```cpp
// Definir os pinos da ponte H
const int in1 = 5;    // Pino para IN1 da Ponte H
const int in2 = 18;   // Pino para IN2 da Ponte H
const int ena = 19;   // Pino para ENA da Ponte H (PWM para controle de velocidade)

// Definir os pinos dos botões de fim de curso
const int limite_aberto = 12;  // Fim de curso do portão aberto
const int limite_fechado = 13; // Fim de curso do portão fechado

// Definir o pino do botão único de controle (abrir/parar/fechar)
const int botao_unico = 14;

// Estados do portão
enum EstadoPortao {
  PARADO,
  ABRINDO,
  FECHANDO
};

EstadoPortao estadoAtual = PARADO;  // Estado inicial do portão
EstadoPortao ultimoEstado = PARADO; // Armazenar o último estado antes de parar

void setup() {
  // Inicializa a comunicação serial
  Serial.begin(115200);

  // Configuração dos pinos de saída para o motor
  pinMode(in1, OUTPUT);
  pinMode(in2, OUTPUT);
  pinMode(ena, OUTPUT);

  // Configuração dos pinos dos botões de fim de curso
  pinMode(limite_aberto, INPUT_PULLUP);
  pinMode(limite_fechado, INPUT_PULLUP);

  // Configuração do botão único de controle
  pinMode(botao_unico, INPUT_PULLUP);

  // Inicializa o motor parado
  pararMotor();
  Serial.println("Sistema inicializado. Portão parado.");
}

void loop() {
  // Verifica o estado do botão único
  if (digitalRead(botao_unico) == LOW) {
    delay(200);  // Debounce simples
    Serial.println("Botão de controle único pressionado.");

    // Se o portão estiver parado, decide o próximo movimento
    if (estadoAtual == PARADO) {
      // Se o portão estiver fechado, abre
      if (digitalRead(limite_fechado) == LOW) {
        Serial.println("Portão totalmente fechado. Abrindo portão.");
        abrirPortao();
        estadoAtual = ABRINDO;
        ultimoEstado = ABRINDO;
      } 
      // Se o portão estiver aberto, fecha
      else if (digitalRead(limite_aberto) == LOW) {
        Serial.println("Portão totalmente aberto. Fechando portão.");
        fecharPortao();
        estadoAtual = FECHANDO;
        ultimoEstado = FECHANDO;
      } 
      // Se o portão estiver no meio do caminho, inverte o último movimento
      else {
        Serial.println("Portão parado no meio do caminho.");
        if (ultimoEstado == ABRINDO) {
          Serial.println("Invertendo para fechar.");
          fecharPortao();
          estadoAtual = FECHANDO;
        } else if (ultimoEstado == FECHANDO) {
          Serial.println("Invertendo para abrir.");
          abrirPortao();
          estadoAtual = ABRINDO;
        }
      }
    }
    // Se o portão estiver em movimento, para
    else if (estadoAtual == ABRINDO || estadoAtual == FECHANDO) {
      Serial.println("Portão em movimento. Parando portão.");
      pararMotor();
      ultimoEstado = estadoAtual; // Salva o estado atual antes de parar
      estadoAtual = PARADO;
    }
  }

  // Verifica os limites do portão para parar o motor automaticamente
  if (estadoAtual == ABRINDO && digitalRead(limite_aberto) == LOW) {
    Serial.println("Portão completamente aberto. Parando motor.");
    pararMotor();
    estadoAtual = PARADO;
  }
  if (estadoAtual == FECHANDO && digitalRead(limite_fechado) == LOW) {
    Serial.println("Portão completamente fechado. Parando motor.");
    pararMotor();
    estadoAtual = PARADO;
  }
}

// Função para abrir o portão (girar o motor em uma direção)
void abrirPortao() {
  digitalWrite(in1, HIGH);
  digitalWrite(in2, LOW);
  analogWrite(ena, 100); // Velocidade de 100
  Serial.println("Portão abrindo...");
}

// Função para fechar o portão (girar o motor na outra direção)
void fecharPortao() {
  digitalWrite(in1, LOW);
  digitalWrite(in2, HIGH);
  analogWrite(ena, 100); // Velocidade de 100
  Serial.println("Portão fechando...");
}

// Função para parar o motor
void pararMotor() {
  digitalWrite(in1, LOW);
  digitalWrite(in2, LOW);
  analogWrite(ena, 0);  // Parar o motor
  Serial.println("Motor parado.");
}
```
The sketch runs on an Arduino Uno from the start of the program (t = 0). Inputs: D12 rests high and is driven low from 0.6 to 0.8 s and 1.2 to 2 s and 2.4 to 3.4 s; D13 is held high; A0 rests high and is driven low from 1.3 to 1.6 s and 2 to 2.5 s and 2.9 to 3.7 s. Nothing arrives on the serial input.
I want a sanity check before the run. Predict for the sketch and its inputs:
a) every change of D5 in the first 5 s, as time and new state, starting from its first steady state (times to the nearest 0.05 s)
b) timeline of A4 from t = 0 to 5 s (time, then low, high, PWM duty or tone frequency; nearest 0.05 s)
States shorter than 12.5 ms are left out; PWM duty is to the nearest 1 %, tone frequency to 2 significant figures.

0 s low; 2.2 s high; 2.4 s low; 3.7 s high
0 s low; 1.5 s high; 1.7 s low; 2.6 s high; 3.1 s low; 3.3 s high; 3.5 s low
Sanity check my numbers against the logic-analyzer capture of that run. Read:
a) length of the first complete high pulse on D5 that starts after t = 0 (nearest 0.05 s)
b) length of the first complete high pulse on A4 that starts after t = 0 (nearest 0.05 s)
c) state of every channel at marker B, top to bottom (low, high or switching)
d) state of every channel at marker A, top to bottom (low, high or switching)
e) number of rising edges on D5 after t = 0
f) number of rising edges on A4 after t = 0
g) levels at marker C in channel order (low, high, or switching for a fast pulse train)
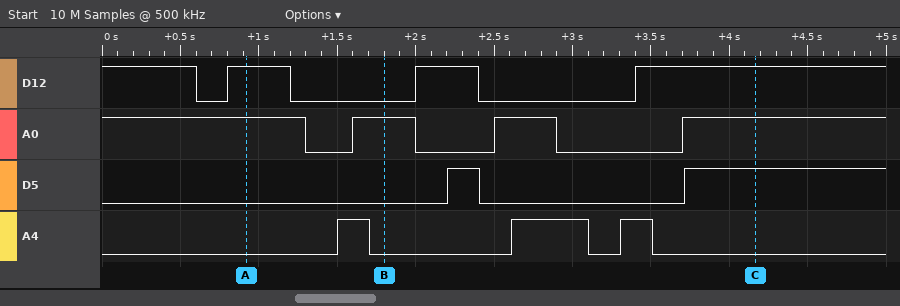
0.20 s
0.20 s
D12 low, A0 high, D5 low, A4 low
D12 high, A0 high, D5 low, A4 low
2
3
D12 high, A0 high, D5 high, A4 low
